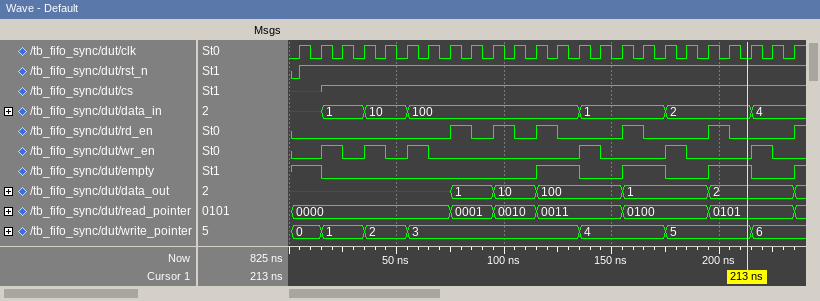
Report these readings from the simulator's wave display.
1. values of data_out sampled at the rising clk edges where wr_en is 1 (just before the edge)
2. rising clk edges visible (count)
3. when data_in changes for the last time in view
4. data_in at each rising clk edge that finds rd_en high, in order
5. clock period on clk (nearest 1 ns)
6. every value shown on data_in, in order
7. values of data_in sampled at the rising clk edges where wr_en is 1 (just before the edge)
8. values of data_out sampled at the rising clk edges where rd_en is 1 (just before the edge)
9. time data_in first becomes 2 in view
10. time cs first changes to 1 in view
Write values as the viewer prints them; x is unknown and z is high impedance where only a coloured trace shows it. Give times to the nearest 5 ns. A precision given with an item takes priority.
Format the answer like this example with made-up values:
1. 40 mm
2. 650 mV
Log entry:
1. x, x, x, 100, 1, 2
2. 24
3. 215 ns
4. 100, 100, 100, 1, 2
5. 10 ns
6. x, 1, 10, 100, 1, 2, 4
7. 1, 10, 100, 1, 2, 4
8. 1, 10, 100, 1, 2
9. 175 ns
10. 15 ns
